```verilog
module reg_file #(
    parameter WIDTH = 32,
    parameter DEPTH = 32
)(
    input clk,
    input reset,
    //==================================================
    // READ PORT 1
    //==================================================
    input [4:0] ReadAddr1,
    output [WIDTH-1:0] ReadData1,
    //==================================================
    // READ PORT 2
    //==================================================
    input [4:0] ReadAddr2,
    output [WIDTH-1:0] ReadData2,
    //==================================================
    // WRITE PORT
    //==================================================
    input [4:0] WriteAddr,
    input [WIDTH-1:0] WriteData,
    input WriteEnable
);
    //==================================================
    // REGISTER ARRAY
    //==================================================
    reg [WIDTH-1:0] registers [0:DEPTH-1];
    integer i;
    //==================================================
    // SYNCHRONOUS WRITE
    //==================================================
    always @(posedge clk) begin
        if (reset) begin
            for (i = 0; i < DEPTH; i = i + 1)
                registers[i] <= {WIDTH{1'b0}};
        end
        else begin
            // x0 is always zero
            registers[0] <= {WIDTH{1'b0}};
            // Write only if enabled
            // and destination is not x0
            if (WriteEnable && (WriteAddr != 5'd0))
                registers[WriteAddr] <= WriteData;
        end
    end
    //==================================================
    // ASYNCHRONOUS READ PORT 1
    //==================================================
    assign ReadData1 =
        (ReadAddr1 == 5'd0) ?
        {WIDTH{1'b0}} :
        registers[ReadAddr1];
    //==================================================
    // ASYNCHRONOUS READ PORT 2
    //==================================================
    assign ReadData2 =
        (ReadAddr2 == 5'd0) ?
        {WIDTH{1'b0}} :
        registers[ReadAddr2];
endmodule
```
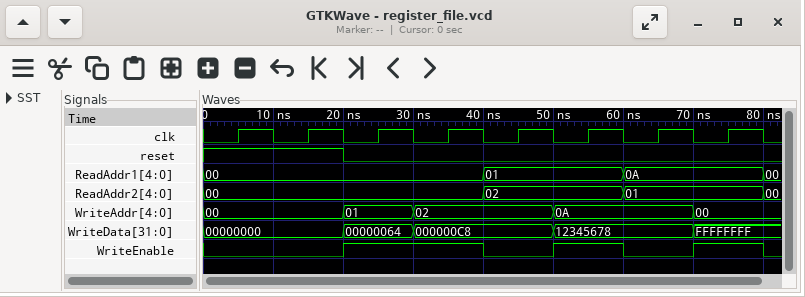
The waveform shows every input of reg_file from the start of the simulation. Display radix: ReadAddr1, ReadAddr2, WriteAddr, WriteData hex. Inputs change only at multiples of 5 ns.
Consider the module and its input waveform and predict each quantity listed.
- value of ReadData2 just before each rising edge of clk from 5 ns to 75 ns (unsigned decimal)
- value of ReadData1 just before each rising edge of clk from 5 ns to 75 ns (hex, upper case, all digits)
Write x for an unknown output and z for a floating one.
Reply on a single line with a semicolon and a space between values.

0, 0, 0, 0, 200, 200, 100, 100; 00000000, 00000000, 00000000, 00000000, 00000064, 00000064, 12345678, 12345678
